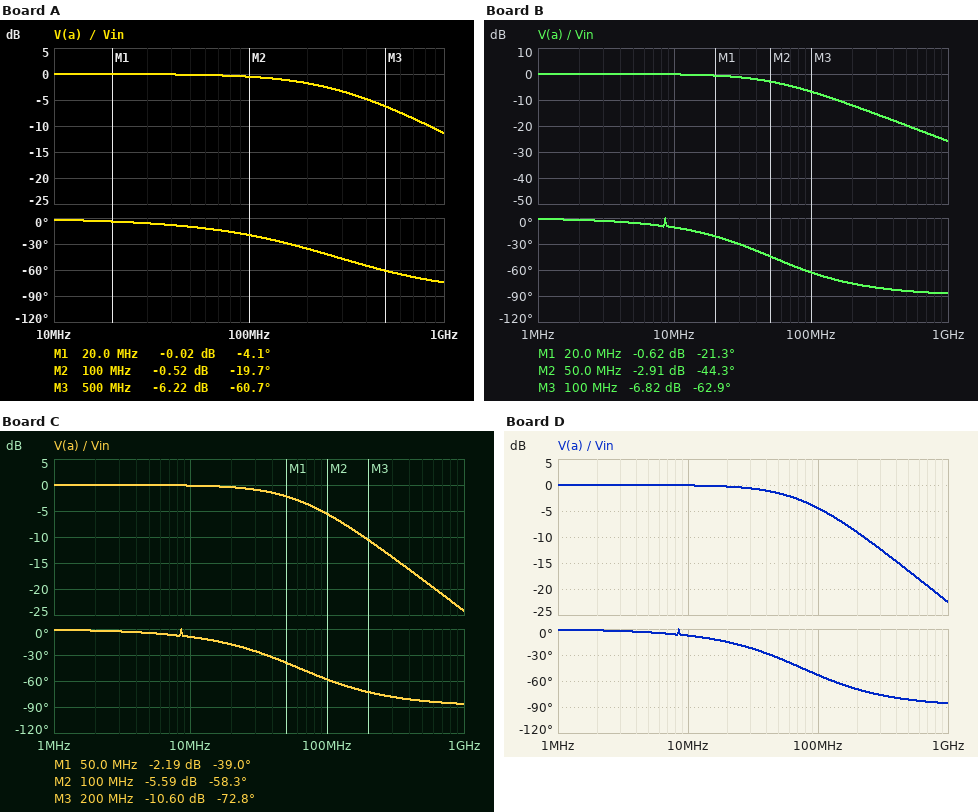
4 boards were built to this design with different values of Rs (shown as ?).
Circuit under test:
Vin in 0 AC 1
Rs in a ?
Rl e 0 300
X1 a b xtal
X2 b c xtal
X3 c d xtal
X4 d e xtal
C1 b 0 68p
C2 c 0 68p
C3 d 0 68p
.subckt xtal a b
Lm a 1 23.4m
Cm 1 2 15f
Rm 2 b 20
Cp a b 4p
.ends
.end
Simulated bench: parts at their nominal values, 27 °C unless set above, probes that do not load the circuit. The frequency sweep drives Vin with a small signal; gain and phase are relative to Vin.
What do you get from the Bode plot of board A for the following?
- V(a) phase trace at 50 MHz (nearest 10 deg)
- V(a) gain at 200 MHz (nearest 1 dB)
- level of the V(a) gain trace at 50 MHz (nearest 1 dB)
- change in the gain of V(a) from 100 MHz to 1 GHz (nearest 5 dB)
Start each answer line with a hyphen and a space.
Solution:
- -10 deg
- -2 dB
- 0 dB
- -10 dB
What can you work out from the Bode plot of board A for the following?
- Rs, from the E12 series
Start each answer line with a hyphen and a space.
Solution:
- 150 Ω
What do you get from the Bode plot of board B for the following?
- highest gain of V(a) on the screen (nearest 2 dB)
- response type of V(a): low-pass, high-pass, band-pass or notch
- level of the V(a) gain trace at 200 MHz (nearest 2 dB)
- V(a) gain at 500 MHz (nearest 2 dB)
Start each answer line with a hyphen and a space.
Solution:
- 0 dB
- low-pass
- -12 dB
- -20 dB
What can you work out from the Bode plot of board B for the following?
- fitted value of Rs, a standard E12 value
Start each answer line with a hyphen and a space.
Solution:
- 820 Ω
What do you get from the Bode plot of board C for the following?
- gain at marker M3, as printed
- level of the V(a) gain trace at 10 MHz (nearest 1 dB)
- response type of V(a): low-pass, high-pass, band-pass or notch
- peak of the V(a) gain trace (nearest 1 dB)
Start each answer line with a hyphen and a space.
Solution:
- -10.60 dB
- 0 dB
- low-pass
- 0 dB
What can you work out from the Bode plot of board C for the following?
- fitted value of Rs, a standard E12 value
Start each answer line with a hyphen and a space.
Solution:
- 680 Ω
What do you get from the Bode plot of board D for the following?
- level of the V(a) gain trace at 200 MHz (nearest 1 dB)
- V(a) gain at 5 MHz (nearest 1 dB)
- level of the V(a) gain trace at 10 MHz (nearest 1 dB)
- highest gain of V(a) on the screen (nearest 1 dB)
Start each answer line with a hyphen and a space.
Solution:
- -9 dB
- 0 dB
- 0 dB
- 0 dB
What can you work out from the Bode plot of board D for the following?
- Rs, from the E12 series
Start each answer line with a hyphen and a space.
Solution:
- 560 Ω
